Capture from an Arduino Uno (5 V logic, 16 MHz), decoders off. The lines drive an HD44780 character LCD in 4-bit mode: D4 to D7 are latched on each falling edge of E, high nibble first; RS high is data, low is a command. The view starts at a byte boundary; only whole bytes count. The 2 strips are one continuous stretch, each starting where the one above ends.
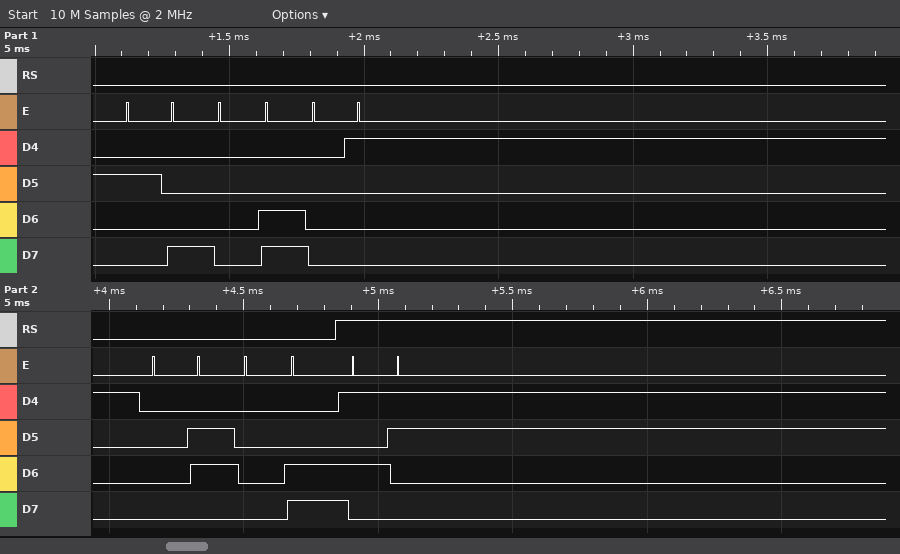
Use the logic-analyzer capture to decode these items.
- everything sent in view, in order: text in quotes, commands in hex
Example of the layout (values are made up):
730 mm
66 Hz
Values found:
0x28 0x0C 0x01 0x06 0x0C "S"
